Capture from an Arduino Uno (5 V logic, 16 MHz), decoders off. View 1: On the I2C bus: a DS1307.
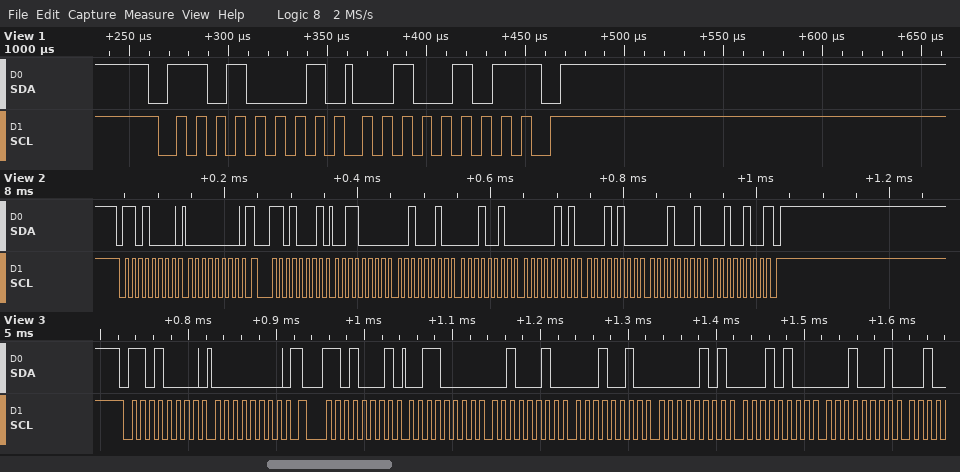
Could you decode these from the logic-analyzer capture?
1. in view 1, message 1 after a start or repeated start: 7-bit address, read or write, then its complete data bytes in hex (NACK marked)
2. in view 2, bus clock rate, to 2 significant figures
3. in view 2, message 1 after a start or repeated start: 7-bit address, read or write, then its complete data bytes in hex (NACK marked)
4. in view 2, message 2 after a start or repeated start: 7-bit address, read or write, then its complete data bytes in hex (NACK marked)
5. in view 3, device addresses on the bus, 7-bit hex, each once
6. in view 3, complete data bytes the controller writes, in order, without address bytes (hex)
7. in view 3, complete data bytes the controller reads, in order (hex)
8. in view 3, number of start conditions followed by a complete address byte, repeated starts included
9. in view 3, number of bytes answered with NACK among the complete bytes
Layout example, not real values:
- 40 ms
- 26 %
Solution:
- 0x68 read: 25 NACK
- 100 kHz
- 0x68 write: 00
- 0x68 read: 30 22 12 05 14 11 24 NACK
- 0x68
- 00
- 30 22 12 05 14 11
- 2
- 0
